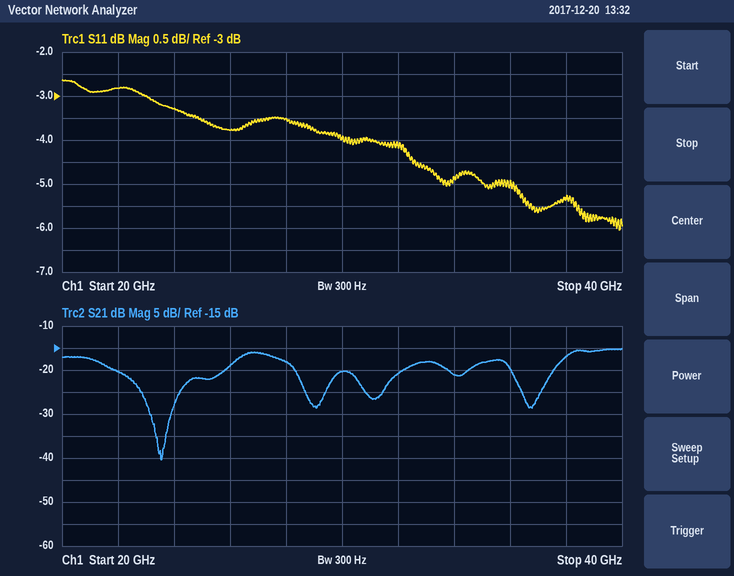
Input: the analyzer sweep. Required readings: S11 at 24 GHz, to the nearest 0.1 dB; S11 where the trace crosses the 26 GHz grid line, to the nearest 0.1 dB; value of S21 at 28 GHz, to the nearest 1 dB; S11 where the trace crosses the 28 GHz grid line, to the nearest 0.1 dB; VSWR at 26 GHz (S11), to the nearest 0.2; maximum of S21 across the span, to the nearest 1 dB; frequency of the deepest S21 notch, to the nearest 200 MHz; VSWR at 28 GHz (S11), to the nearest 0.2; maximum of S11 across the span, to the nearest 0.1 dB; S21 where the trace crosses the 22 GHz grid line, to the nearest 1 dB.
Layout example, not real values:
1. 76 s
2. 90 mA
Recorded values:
1. -3.3 dB
2. -3.8 dB
3. -18 dB
4. -3.5 dB
5. 4.6
6. -15 dB
7. 23.6 GHz
8. 5.0
9. -2.6 dB
10. -20 dB
